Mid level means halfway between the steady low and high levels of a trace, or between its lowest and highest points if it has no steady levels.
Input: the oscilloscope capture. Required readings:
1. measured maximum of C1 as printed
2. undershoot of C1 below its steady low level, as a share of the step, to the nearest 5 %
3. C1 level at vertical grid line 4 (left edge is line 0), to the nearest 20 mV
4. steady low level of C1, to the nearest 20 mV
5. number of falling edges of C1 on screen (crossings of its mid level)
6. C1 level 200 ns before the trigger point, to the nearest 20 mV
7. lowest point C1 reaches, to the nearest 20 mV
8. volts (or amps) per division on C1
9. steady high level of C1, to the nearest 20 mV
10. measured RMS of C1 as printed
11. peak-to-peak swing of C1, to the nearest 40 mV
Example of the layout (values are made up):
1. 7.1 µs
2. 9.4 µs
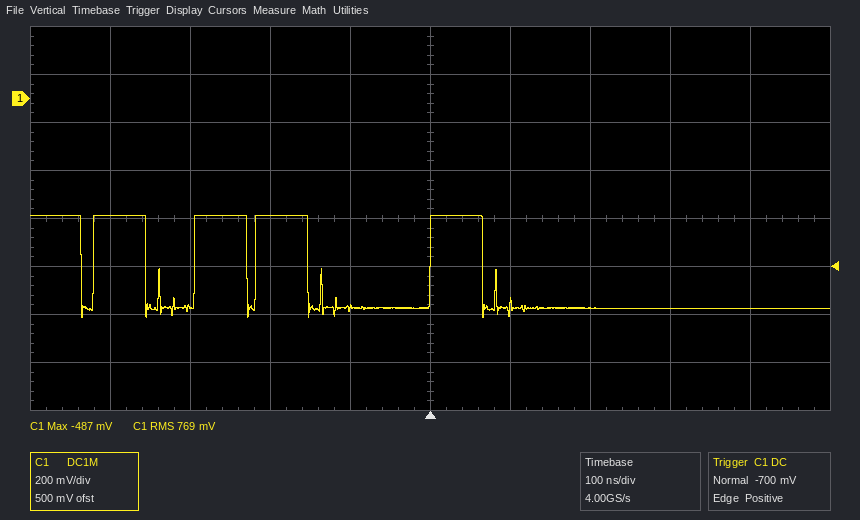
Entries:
1. -487 mV
2. 10 %
3. -880 mV
4. -880 mV
5. 5
6. -480 mV
7. -920 mV
8. 200 mV
9. -480 mV
10. 769 mV
11. 440 mV
